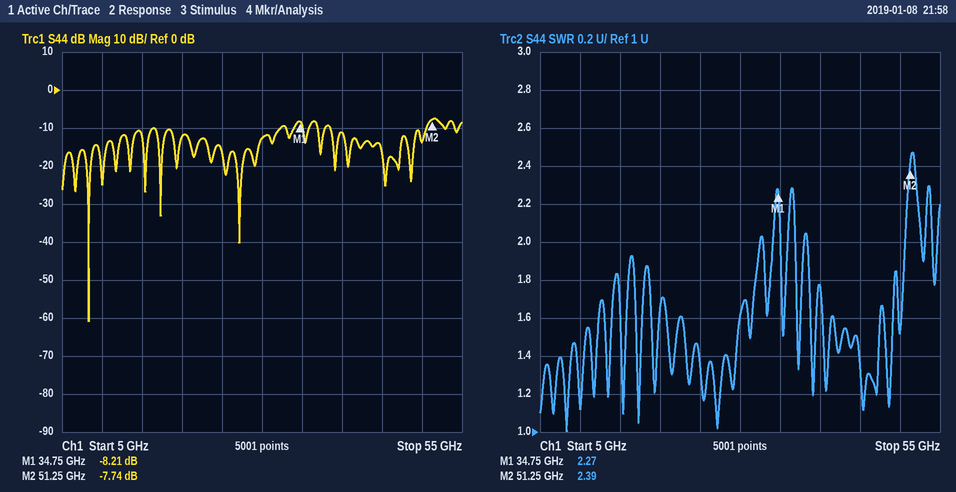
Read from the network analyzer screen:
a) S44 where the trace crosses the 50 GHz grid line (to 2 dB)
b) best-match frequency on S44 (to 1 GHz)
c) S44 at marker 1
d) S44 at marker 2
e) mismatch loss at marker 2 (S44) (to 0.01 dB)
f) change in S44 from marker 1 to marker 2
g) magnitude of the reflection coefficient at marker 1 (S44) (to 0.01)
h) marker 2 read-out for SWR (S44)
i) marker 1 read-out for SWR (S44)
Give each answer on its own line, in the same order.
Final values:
-14 dB
8 GHz
-8.21 dB
-7.74 dB
0.80 dB
0.47 dB
0.39
2.39
2.27
